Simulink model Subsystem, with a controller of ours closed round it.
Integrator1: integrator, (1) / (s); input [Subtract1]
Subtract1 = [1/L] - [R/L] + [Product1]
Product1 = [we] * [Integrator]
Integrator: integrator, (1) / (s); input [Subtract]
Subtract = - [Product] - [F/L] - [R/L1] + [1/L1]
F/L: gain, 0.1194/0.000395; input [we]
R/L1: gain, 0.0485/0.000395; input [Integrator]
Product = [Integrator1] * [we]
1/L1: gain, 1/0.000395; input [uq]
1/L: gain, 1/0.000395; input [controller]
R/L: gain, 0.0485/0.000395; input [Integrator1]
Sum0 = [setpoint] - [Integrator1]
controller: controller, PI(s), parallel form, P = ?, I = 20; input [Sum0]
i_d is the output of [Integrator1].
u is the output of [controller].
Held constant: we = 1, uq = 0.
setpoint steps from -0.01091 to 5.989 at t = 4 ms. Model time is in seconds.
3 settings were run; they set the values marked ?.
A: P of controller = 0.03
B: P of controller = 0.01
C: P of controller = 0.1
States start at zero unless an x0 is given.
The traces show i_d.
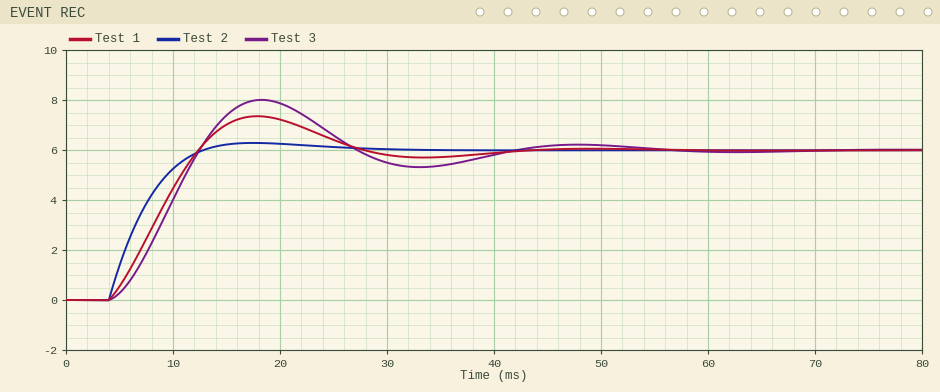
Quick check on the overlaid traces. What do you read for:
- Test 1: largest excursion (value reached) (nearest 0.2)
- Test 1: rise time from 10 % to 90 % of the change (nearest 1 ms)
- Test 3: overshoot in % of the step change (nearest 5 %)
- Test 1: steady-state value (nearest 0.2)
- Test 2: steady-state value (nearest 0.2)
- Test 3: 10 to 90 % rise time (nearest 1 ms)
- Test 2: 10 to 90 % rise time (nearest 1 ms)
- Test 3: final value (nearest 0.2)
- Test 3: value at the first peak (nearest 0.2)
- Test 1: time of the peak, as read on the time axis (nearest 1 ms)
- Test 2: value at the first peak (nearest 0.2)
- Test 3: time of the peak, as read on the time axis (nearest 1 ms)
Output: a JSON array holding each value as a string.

["7.4", "6 ms", "35 %", "6.0", "6.0", "6 ms", "6 ms", "6.0", "8.0", "18 ms", "6.2", "18 ms"]
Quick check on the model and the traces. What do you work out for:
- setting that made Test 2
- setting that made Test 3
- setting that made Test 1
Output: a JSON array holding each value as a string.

["C", "B", "A"]
